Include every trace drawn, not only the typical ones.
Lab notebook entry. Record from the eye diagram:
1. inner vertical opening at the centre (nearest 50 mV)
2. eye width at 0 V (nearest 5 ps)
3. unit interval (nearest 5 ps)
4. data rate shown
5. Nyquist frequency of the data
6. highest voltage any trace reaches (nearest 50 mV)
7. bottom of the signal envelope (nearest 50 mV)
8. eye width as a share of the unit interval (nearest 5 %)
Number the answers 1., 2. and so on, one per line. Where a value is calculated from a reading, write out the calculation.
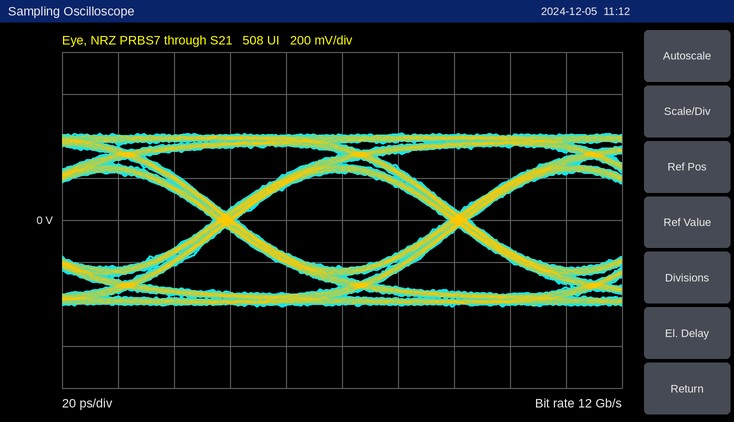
1. 450 mV
2. 75 ps
3. 85 ps
4. 12 Gb/s
5. 6 GHz
6. 400 mV
7. -400 mV
8. 75 ps / 85 ps ≈ 88.2 %, so 90 % to the nearest 5 %
